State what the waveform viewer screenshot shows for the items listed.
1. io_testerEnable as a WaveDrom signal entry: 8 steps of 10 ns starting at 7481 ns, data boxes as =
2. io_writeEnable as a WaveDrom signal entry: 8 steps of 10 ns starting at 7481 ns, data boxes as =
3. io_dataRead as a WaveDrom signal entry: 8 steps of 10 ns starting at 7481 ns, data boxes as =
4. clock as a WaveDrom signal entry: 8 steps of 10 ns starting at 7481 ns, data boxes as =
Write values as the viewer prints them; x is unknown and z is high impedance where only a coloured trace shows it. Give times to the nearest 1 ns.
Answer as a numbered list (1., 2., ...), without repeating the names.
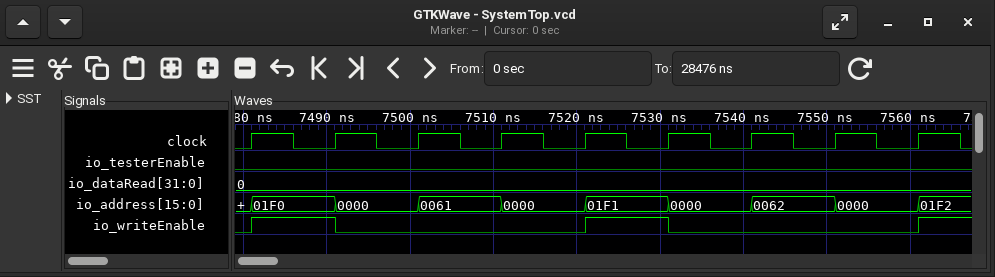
1. {name: 'io_testerEnable', wave: '0.......'}
2. {name: 'io_writeEnable', wave: '10..10..'}
3. {name: 'io_dataRead', wave: '=.......', data: '0'}
4. {name: 'clock', wave: 'p.......'}
